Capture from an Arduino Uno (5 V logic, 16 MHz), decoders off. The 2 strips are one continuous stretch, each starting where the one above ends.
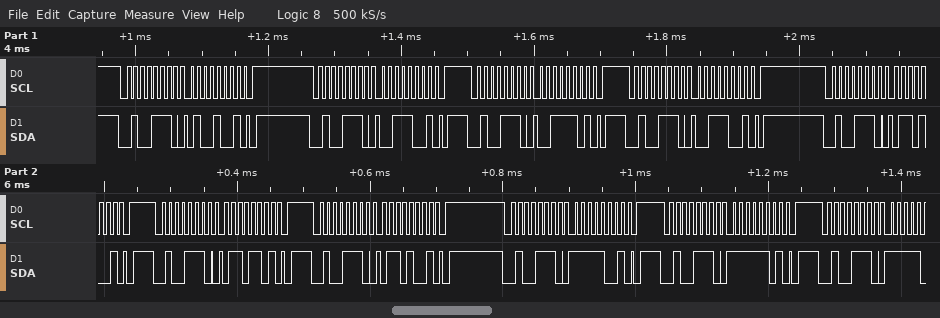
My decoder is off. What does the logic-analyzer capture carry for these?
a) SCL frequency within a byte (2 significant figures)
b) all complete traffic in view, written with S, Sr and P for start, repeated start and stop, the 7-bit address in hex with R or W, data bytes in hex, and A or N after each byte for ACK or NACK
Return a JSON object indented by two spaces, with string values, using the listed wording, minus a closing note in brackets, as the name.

{
  "SCL frequency within a byte": "100 kHz",
  "all complete traffic in view, written with S, Sr and P for start, repeated start and stop, the 7-bit address in hex with R or W, data bytes in hex, and A or N after each byte for ACK or NACK": "S 27W A 49 A P S 27W A 39 A P S 27W A 3D A P S 27W A 39 A P S 27W A 69 A P S 27W A 6D A P S 27W A 69 A P S 27W A F9 A P S 27W A FD A P S 27W A"
}
